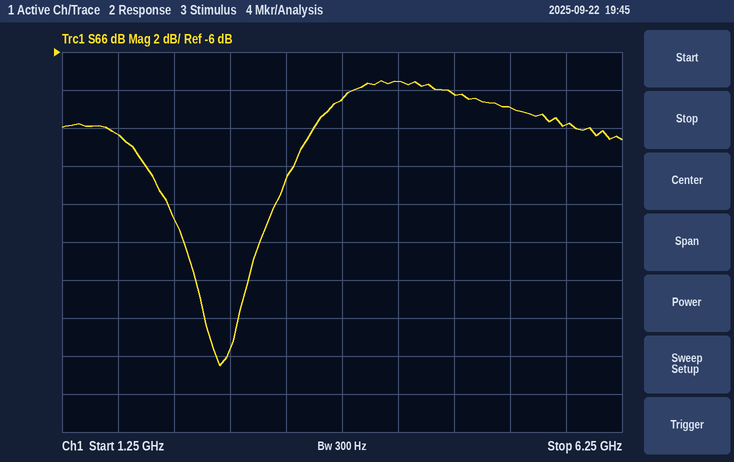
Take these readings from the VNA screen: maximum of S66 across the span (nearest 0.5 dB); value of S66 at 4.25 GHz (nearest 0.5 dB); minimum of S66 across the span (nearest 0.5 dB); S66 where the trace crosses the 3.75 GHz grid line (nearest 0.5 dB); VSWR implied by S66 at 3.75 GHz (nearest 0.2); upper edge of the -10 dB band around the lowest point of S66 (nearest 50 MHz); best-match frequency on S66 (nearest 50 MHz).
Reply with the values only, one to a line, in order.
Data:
-7.5 dB
-7.5 dB
-22.5 dB
-8.5 dB
2.2
3.50 GHz
2.65 GHz
